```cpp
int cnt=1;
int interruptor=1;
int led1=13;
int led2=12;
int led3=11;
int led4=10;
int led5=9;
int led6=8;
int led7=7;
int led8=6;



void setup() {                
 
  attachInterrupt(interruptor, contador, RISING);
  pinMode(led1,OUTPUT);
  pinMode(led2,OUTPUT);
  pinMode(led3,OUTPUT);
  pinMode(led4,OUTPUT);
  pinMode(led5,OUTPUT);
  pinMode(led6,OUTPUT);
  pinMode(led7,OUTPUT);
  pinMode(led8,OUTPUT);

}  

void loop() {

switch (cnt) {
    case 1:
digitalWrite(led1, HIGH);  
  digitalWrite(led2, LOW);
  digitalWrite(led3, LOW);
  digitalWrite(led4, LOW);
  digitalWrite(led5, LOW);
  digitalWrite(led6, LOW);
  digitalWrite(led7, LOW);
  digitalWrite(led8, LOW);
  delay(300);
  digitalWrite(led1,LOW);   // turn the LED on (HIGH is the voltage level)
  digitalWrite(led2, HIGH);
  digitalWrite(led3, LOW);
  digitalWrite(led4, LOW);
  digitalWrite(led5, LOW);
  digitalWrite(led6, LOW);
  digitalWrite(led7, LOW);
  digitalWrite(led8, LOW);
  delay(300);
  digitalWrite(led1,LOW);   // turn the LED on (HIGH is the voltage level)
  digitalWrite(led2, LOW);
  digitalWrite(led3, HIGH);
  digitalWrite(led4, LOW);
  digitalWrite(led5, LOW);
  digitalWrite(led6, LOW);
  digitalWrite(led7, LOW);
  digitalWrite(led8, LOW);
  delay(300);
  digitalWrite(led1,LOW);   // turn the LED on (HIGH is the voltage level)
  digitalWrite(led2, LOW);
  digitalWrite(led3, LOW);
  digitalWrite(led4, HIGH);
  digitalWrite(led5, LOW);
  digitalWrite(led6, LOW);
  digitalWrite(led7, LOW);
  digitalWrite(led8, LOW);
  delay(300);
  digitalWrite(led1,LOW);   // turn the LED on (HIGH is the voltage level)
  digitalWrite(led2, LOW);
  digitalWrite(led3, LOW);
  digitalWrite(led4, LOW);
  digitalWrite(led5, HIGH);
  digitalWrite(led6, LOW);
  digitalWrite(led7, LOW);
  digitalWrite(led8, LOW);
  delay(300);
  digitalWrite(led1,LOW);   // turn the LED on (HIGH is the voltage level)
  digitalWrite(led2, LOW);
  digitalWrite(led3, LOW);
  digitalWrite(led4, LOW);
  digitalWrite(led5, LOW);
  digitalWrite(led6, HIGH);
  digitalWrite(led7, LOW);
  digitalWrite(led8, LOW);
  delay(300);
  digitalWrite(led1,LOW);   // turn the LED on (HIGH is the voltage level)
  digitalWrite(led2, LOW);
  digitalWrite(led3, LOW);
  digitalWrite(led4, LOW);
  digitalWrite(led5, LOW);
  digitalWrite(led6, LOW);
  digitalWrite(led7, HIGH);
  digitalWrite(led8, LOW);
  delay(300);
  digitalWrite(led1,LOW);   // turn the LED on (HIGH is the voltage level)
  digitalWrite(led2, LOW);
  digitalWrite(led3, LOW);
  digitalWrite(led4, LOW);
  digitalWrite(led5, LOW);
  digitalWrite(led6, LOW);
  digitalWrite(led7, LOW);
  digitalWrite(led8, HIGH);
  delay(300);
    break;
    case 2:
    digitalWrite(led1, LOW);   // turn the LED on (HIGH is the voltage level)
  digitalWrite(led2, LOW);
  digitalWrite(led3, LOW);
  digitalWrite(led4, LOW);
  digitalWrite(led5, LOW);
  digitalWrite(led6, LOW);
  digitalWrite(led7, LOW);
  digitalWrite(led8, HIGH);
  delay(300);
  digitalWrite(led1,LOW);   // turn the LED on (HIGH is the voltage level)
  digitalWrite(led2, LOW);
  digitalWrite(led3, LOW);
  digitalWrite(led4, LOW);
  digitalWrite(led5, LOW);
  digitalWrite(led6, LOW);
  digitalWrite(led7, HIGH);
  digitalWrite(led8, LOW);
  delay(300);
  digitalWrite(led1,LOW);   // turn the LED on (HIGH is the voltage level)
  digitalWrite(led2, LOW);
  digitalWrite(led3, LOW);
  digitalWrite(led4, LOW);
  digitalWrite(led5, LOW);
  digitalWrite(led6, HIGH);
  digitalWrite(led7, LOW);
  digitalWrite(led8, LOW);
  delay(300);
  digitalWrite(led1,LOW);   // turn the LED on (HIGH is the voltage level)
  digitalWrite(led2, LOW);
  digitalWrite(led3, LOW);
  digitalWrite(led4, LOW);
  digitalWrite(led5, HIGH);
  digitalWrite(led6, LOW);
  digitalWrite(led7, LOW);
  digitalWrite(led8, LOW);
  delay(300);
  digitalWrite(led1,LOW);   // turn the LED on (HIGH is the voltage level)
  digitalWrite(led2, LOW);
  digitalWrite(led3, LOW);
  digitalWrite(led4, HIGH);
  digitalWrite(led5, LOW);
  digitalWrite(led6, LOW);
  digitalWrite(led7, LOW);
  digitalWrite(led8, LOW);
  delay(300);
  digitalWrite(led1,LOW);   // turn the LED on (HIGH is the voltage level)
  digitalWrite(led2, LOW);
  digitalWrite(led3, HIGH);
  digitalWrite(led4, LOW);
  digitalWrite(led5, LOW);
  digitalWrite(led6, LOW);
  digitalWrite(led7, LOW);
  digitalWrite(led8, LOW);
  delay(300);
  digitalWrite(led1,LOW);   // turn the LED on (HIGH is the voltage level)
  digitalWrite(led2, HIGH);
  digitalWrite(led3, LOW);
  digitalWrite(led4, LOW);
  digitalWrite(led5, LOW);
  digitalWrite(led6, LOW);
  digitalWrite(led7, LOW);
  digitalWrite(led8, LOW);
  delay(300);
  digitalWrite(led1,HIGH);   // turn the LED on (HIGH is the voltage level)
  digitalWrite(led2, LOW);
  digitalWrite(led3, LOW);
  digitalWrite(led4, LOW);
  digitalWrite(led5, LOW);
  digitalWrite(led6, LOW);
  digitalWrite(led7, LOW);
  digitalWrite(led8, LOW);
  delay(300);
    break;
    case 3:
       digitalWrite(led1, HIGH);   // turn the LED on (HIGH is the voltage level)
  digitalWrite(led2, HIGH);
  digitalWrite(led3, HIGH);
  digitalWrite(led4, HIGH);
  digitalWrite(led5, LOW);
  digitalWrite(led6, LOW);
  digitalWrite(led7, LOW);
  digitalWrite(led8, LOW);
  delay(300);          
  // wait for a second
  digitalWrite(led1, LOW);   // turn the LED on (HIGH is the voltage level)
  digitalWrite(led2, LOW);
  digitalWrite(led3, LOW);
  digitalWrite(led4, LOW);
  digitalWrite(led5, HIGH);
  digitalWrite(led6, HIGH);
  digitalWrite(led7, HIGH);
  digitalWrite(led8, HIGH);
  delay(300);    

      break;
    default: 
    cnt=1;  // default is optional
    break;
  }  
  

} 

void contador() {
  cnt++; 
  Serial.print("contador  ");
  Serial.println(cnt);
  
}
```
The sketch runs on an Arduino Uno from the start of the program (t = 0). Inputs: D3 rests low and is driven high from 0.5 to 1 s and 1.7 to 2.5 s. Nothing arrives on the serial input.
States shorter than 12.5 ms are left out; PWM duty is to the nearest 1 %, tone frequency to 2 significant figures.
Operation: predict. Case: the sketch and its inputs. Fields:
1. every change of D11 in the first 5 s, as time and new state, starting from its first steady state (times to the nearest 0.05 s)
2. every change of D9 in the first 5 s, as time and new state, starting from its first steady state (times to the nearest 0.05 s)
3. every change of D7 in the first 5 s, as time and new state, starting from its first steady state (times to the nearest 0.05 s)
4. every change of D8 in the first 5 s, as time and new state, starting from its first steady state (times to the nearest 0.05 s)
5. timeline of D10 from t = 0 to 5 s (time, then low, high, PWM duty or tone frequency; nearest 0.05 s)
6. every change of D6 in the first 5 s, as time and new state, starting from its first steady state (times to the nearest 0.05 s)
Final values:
0 s low; 0.6 s high; 0.9 s low; 2.4 s high; 2.7 s low; 3 s high; 3.3 s low; 3.6 s high; 3.9 s low; 4.2 s high; 4.5 s low; 4.8 s high
0 s low; 1.2 s high; 1.5 s low; 2.7 s high; 3 s low; 3.3 s high; 3.6 s low; 3.9 s high; 4.2 s low; 4.5 s high; 4.8 s low
0 s low; 1.8 s high; 2.1 s low; 2.7 s high; 3 s low; 3.3 s high; 3.6 s low; 3.9 s high; 4.2 s low; 4.5 s high; 4.8 s low
0 s low; 1.5 s high; 1.8 s low; 2.7 s high; 3 s low; 3.3 s high; 3.6 s low; 3.9 s high; 4.2 s low; 4.5 s high; 4.8 s low
0 s low; 0.9 s high; 1.2 s low; 2.4 s high; 2.7 s low; 3 s high; 3.3 s low; 3.6 s high; 3.9 s low; 4.2 s high; 4.5 s low; 4.8 s high
0 s low; 2.1 s high; 2.4 s low; 2.7 s high; 3 s low; 3.3 s high; 3.6 s low; 3.9 s high; 4.2 s low; 4.5 s high; 4.8 s low
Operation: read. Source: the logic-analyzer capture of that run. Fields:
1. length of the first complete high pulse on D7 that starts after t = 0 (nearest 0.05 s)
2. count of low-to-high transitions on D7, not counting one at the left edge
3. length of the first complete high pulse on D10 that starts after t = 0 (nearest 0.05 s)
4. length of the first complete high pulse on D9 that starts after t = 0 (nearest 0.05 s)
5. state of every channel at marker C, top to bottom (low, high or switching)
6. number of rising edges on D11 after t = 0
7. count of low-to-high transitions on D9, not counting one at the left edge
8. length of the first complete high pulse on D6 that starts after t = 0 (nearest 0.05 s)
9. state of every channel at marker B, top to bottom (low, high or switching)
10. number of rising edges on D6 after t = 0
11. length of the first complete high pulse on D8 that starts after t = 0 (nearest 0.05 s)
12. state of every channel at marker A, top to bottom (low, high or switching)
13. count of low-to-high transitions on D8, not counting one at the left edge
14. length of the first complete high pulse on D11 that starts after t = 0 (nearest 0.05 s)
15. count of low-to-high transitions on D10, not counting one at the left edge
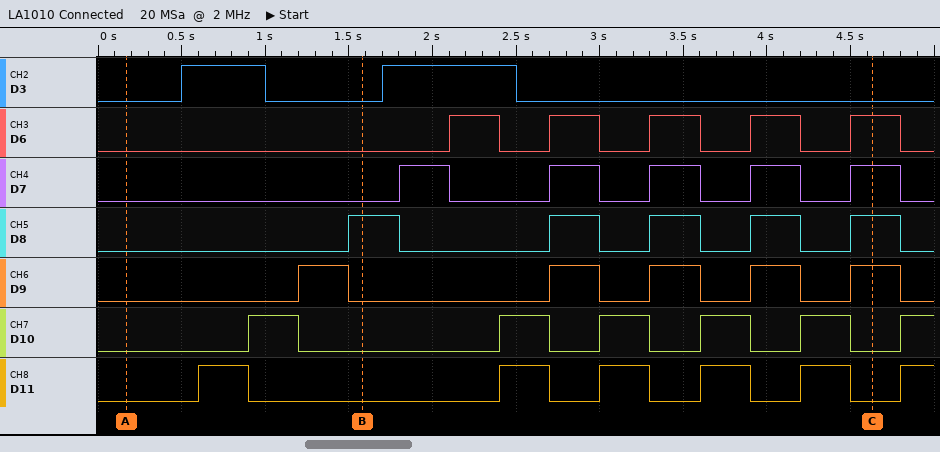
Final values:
0.30 s
5
0.30 s
0.30 s
D3 low, D6 high, D7 high, D8 high, D9 high, D10 low, D11 low
6
5
0.30 s
D3 low, D6 low, D7 low, D8 high, D9 low, D10 low, D11 low
5
0.30 s
D3 low, D6 low, D7 low, D8 low, D9 low, D10 low, D11 low
5
0.30 s
6
